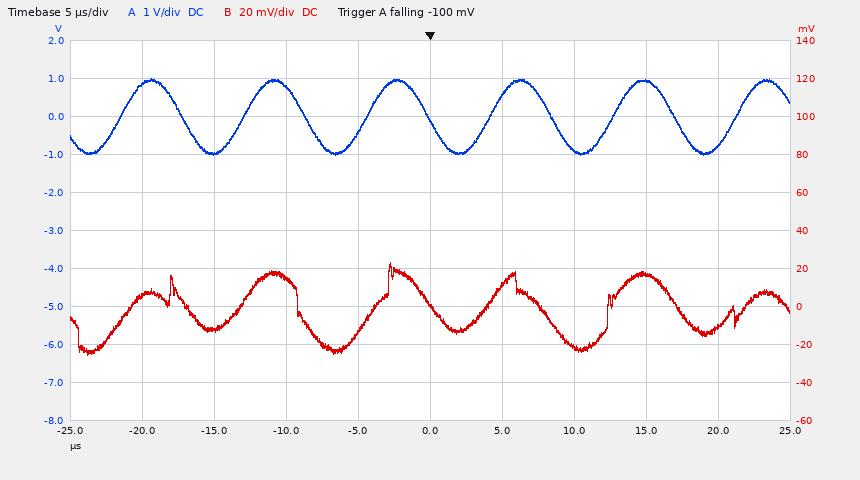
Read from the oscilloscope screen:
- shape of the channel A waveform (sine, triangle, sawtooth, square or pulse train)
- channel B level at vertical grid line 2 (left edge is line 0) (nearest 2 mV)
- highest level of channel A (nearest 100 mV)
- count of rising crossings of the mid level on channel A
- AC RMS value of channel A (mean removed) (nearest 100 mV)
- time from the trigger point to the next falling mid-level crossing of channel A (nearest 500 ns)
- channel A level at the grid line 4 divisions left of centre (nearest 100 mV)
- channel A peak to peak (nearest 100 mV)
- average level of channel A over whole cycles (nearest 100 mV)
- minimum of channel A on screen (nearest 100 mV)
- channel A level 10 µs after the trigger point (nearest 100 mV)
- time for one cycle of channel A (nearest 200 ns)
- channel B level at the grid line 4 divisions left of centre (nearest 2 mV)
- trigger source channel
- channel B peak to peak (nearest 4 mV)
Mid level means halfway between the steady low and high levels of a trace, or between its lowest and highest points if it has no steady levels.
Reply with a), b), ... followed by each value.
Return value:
a) sine
b) -12 mV
c) 1.0 V
d) 6
e) 700 mV
f) 8.5 µs
g) 900 mV
h) 2.0 V
i) 0.0 V
j) -1.0 V
k) -900 mV
l) 8.6 µs
m) 6 mV
n) channel A
o) 48 mV
